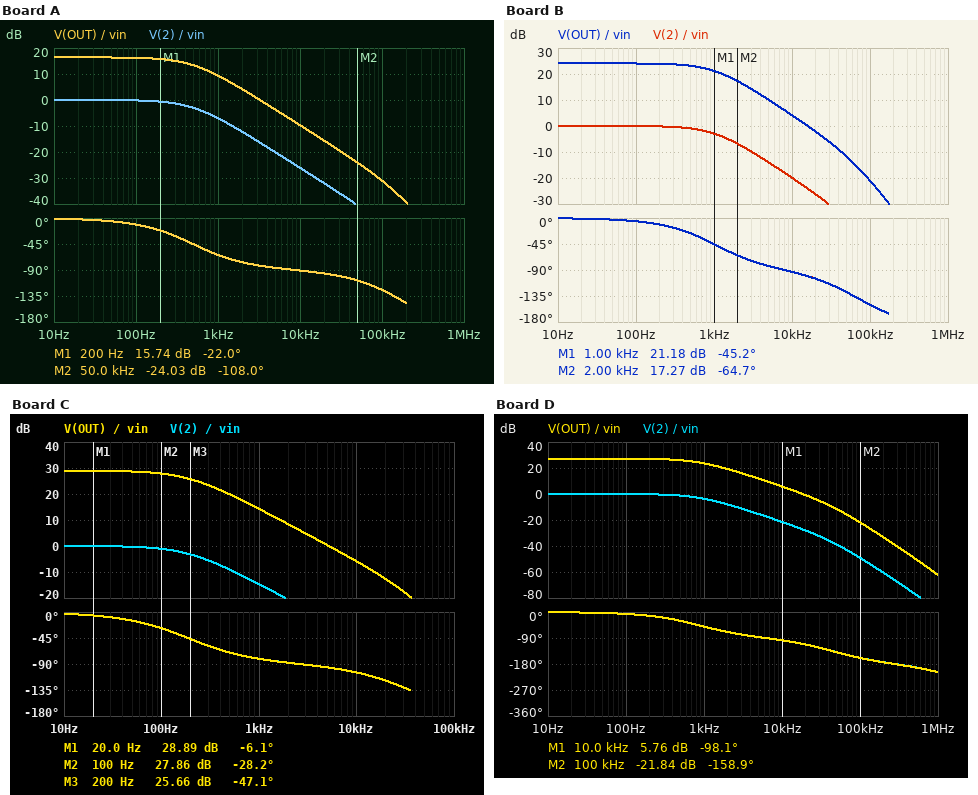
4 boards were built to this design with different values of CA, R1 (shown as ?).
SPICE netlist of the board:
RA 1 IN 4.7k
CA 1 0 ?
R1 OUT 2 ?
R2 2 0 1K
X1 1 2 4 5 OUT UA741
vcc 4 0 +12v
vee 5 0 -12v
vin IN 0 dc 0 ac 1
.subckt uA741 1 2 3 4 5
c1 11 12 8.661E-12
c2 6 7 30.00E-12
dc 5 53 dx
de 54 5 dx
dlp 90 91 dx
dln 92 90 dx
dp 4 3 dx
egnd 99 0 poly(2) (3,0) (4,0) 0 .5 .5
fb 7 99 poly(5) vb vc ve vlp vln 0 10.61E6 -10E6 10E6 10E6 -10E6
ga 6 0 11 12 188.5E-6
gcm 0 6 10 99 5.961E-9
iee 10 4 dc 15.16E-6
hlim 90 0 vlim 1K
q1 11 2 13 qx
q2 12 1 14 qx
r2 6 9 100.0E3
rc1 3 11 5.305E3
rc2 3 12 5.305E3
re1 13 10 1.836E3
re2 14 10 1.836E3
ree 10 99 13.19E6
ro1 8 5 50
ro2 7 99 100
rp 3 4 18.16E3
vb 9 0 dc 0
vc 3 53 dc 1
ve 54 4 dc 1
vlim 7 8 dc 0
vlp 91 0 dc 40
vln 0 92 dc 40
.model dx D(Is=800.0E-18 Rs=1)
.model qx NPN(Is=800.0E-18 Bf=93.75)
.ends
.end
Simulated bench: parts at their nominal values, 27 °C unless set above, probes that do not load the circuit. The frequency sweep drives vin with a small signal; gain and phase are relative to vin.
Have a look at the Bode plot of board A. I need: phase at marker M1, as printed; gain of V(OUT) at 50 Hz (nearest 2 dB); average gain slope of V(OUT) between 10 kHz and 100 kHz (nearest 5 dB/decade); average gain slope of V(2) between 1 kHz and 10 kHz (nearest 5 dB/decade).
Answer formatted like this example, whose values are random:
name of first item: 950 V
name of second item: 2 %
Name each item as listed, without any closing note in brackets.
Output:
phase at marker M1, as printed: -22.0 deg
gain of V(OUT) at 50 Hz: 16 dB
average gain slope of V(OUT) between 10 kHz and 100 kHz: -20 dB/decade
average gain slope of V(2) between 1 kHz and 10 kHz: -20 dB/decade
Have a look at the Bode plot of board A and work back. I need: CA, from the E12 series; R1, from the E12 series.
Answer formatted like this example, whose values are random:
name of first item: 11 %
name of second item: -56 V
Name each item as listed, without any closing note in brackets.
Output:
CA, from the E12 series: 68 nF
R1, from the E12 series: 5.6 kΩ
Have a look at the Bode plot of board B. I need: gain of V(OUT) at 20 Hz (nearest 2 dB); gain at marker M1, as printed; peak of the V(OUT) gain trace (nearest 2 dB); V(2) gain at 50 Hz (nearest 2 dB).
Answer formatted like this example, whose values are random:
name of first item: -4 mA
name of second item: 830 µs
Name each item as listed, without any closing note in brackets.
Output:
gain of V(OUT) at 20 Hz: 24 dB
gain at marker M1, as printed: 21.18 dB
peak of the V(OUT) gain trace: 24 dB
V(2) gain at 50 Hz: 0 dB
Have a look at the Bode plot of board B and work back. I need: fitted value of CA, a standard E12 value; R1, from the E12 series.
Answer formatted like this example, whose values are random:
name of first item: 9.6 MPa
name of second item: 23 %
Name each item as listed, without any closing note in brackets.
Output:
fitted value of CA, a standard E12 value: 33 nF
R1, from the E12 series: 15 kΩ
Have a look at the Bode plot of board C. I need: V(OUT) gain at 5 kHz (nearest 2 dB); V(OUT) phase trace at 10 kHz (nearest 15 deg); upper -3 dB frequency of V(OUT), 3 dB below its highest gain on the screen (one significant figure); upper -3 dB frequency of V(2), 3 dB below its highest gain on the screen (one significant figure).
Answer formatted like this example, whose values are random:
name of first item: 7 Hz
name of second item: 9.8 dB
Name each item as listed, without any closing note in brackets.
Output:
V(OUT) gain at 5 kHz: 0 dB
V(OUT) phase trace at 10 kHz: -105 deg
upper -3 dB frequency of V(OUT), 3 dB below its highest gain on the screen: 200 Hz
upper -3 dB frequency of V(2), 3 dB below its highest gain on the screen: 200 Hz
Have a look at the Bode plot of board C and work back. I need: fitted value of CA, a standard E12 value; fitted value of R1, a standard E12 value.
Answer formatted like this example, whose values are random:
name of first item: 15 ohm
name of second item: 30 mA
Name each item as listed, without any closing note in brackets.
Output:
fitted value of CA, a standard E12 value: 180 nF
fitted value of R1, a standard E12 value: 27 kΩ
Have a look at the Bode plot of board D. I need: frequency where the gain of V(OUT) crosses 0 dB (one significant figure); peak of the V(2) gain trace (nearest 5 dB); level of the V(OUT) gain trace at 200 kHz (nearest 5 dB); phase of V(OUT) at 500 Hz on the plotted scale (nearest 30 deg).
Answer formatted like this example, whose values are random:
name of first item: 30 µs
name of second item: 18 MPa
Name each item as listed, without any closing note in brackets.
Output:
frequency where the gain of V(OUT) crosses 0 dB: 20 kHz
peak of the V(2) gain trace: 0 dB
level of the V(OUT) gain trace at 200 kHz: -35 dB
phase of V(OUT) at 500 Hz on the plotted scale: -30 deg
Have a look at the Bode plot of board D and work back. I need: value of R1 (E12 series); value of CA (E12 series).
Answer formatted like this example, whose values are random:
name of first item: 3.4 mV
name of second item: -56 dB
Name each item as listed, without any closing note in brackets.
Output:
value of R1: 22 kΩ
value of CA: 39 nF
